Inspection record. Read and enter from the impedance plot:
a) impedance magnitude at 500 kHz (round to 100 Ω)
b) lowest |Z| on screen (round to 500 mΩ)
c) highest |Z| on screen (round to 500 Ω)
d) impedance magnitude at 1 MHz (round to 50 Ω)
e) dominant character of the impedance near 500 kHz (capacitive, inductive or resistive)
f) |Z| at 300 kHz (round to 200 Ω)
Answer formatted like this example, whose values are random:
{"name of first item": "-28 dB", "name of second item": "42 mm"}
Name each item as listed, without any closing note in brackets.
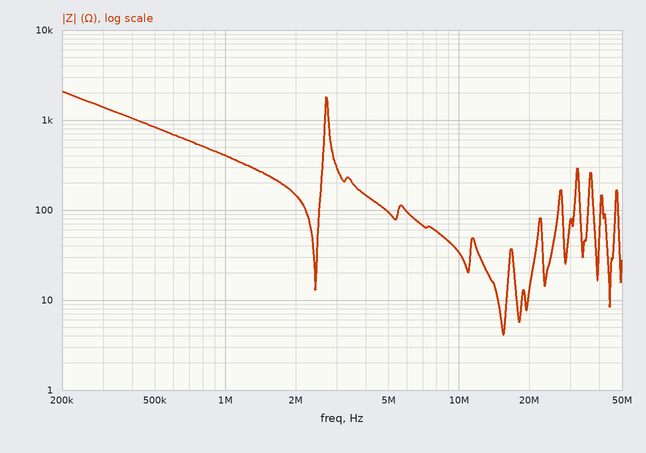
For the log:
{"impedance magnitude at 500 kHz": "800 Ω", "lowest |Z| on screen": "4.0 Ω", "highest |Z| on screen": "2.0 kΩ", "impedance magnitude at 1 MHz": "400 Ω", "dominant character of the impedance near 500 kHz": "capacitive", "|Z| at 300 kHz": "1.4 kΩ"}
